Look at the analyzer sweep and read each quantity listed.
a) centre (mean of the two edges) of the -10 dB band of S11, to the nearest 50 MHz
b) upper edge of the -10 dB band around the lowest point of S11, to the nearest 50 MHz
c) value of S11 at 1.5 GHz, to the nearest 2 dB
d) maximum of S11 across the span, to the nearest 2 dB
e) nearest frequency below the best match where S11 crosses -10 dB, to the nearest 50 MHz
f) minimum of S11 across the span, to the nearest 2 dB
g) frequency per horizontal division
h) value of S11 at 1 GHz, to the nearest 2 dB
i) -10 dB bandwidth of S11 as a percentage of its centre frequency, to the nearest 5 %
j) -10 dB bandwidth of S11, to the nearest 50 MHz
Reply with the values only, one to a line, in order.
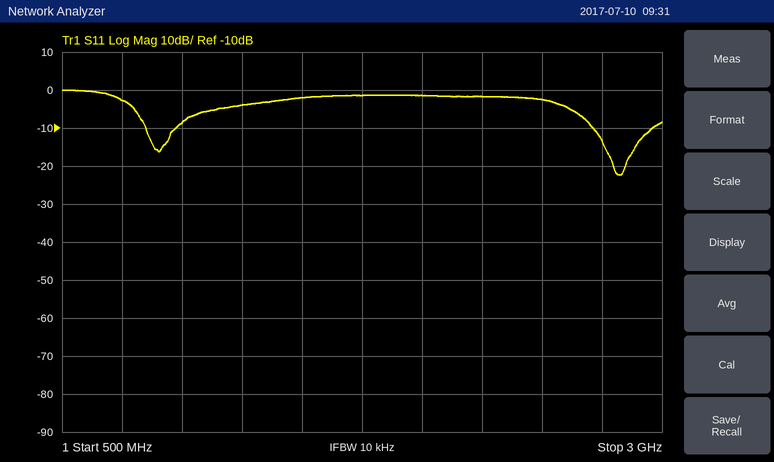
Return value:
2.85 GHz
2.95 GHz
-2 dB
0 dB
2.70 GHz
-22 dB
250 MHz
-8 dB
10 %
250 MHz
